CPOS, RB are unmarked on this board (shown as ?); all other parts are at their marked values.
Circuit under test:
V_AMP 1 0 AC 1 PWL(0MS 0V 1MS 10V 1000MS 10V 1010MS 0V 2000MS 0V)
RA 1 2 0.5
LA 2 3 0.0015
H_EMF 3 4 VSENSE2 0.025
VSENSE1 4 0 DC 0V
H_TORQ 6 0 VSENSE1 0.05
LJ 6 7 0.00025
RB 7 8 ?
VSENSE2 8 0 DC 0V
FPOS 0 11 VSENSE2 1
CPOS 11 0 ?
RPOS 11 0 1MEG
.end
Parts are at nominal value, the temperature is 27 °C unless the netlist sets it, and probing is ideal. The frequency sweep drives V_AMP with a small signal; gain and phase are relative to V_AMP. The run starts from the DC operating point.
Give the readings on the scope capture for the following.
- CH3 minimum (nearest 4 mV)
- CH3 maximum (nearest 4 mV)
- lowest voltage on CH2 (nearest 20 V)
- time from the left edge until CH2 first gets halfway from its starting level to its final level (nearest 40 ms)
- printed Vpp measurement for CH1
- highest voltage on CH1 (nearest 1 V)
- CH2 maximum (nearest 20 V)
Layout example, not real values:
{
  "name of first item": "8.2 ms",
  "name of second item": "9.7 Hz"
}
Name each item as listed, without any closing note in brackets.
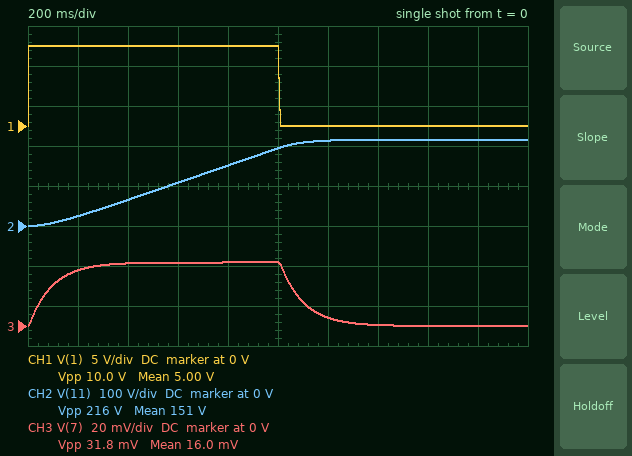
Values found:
{
  "CH3 minimum": "0 V",
  "CH3 maximum": "32 mV",
  "lowest voltage on CH2": "0 V",
  "time from the left edge until CH2 first gets halfway from its starting level to its final level": "600 ms",
  "printed Vpp measurement for CH1": "10.0 V",
  "highest voltage on CH1": "10 V",
  "CH2 maximum": "220 V"
}
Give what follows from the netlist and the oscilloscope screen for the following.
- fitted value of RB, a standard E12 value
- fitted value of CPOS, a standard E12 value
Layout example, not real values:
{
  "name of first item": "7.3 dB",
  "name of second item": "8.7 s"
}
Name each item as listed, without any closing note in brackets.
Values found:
{
  "fitted value of RB, a standard E12 value": "82 µΩ",
  "fitted value of CPOS, a standard E12 value": "1.8 F"
}
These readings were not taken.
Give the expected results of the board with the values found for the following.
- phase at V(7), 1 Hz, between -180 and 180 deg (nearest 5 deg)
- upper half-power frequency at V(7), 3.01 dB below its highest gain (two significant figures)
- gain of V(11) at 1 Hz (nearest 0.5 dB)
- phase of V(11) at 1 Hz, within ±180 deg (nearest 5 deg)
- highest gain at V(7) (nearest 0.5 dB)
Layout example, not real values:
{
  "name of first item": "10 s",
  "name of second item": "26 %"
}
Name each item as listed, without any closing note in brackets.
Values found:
{
  "phase at V(7), 1 Hz, between -180 and 180 deg": "-30 deg",
  "upper half-power frequency at V(7), 3.01 dB below its highest gain": "1.7 Hz",
  "gain of V(11) at 1 Hz": "9.5 dB",
  "phase of V(11) at 1 Hz, within ±180 deg": "-120 deg",
  "highest gain at V(7)": "-50.0 dB"
}
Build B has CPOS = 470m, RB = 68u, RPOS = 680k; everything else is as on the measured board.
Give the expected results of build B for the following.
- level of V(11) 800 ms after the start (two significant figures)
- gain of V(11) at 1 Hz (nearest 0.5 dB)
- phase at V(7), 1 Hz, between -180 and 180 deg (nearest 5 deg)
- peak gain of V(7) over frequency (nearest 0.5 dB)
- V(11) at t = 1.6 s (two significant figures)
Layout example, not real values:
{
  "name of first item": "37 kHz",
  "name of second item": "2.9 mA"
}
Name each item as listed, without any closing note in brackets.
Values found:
{
  "level of V(11) 800 ms after the start": "580 V",
  "gain of V(11) at 1 Hz": "21.0 dB",
  "phase at V(7), 1 Hz, between -180 and 180 deg": "-30 deg",
  "peak gain of V(7) over frequency": "-51.5 dB",
  "V(11) at t = 1.6 s": "830 V"
}
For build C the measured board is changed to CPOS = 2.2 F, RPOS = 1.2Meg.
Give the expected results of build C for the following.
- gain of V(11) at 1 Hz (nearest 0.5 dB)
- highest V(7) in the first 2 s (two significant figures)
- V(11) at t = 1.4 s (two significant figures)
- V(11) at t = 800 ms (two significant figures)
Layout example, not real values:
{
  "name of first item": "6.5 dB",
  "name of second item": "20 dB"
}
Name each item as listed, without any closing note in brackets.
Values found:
{
  "gain of V(11) at 1 Hz": "7.5 dB",
  "highest V(7) in the first 2 s": "32 mV",
  "V(11) at t = 1.4 s": "180 V",
  "V(11) at t = 800 ms": "120 V"
}
